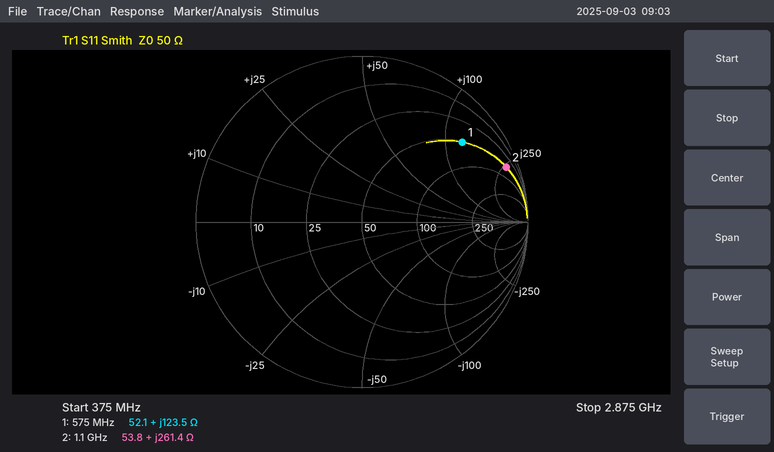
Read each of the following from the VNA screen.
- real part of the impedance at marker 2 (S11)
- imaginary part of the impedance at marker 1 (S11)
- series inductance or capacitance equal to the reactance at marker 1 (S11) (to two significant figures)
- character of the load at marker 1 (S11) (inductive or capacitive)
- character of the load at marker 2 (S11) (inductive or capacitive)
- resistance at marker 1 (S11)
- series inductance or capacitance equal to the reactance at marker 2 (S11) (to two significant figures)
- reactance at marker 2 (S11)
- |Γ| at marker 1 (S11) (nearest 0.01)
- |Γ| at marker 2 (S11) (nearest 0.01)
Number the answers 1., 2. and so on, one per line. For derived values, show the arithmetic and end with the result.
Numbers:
1. 53.8 Ω
2. +123.5 Ω
3. L = 123.5 Ω/(2π × 575 MHz) ≈ 34 nH
4. inductive
5. inductive
6. 52.1 Ω
7. L = 261.4 Ω/(2π × 1.1 GHz) ≈ 38 nH
8. +261.4 Ω
9. 0.77
10. 0.93
